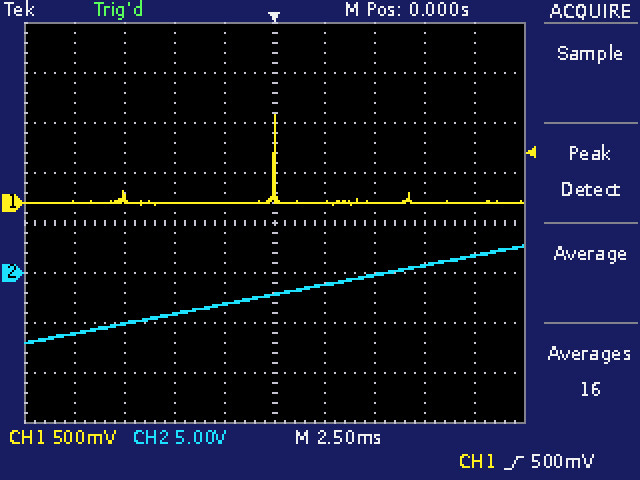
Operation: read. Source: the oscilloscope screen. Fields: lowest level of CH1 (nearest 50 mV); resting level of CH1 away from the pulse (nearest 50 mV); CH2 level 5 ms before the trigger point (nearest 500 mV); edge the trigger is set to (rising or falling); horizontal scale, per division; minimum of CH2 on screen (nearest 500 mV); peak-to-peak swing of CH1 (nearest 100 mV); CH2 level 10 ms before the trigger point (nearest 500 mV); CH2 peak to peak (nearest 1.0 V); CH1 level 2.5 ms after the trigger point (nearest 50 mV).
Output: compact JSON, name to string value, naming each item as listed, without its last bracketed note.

{"lowest level of CH1": "0 mV", "resting level of CH1 away from the pulse": "0 mV", "CH2 level 5 ms before the trigger point": "-4.0 V", "edge the trigger is set to": "rising", "horizontal scale, per division": "2.5 ms", "minimum of CH2 on screen": "-7.0 V", "peak-to-peak swing of CH1": "900 mV", "CH2 level 10 ms before the trigger point": "-6.0 V", "CH2 peak to peak": "10.0 V", "CH1 level 2.5 ms after the trigger point": "0 mV"}
